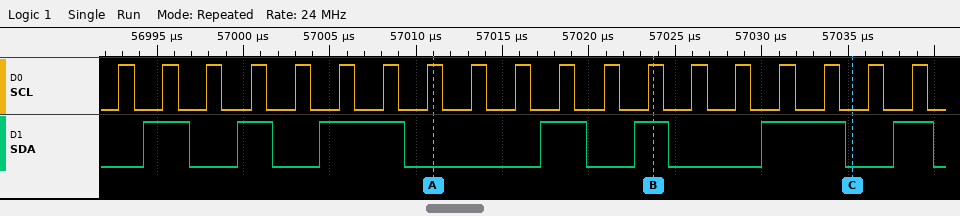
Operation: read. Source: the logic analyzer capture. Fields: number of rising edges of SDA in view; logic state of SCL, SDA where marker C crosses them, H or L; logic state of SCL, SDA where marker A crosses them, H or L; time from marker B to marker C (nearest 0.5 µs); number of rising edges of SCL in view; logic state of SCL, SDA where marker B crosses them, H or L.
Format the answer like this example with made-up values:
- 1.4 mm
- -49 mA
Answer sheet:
- 7
- SCL=L, SDA=L
- SCL=H, SDA=L
- 11.5 µs
- 19
- SCL=H, SDA=H
